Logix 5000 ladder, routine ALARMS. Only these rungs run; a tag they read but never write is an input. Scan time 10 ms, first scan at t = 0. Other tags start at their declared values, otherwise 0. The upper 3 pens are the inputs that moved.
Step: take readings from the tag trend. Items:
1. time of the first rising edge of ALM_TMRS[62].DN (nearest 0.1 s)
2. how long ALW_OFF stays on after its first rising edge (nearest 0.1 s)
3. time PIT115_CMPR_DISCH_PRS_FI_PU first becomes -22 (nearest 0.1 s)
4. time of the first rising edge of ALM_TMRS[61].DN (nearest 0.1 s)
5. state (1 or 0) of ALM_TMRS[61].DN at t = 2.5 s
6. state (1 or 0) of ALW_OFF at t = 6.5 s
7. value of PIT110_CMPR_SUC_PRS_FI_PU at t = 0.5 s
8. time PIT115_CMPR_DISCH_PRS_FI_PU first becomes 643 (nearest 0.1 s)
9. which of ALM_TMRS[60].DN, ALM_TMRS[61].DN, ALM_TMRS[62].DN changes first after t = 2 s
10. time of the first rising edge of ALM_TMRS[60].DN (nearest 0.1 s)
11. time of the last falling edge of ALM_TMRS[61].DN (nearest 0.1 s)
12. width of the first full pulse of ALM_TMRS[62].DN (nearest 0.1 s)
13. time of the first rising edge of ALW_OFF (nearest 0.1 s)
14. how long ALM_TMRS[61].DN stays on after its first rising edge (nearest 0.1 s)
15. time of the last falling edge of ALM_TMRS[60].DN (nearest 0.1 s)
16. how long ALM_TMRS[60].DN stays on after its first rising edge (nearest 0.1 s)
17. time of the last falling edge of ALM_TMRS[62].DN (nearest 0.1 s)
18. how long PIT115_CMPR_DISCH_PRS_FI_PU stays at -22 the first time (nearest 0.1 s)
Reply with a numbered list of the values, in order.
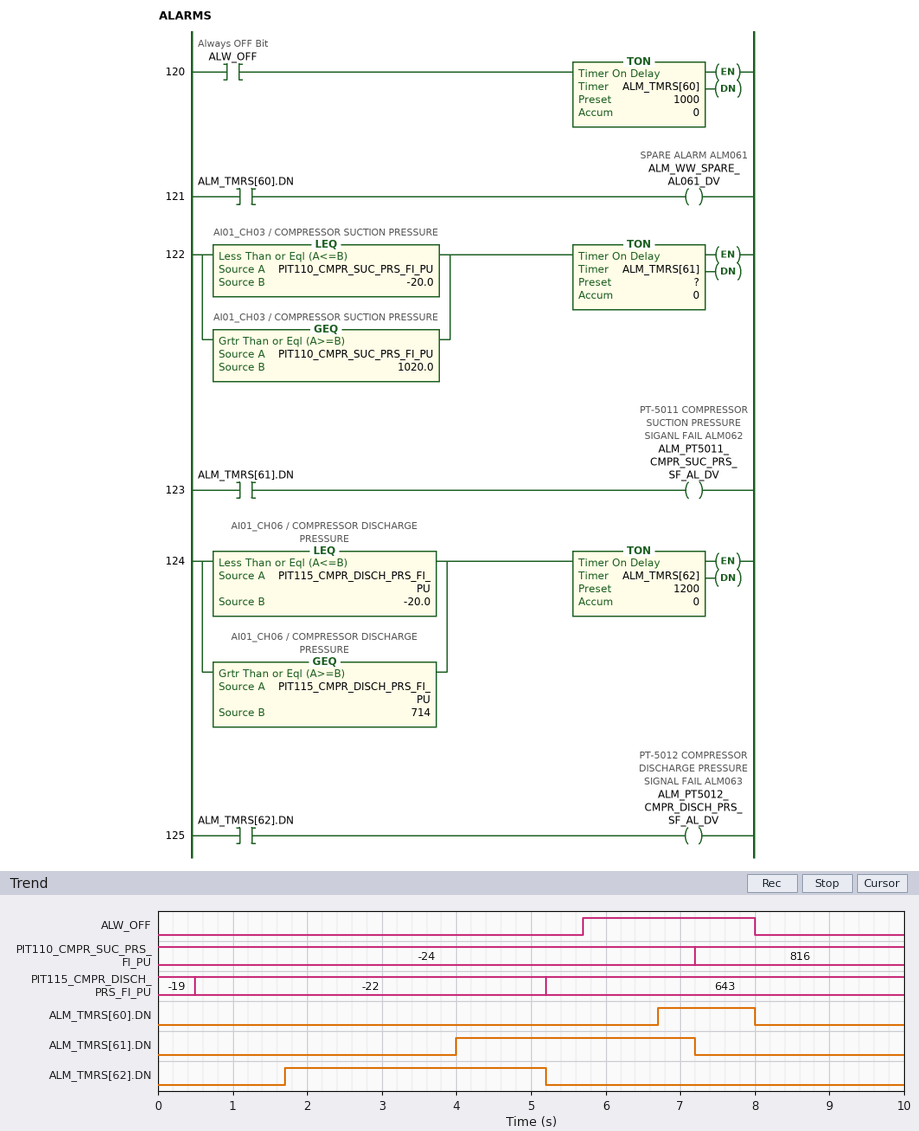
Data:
1. 1.7 s
2. 2.3 s
3. 0.5 s
4. 4.0 s
5. 0
6. 1
7. -24
8. 5.2 s
9. ALM_TMRS[61].DN
10. 6.7 s
11. 7.2 s
12. 3.5 s
13. 5.7 s
14. 3.2 s
15. 8.0 s
16. 1.3 s
17. 5.2 s
18. 4.7 s
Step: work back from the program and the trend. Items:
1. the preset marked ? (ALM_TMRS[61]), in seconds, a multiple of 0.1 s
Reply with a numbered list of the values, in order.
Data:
1. 4.0 s
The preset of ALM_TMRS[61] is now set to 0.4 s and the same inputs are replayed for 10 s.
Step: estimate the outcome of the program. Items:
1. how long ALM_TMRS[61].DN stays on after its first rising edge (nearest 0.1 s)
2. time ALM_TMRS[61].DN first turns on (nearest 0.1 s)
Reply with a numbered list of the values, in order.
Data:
1. 6.8 s
2. 0.4 s
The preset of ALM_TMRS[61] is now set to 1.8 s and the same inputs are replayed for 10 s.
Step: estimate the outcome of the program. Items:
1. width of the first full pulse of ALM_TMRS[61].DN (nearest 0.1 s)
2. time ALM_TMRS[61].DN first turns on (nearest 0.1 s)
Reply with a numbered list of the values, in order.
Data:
1. 5.4 s
2. 1.8 s
